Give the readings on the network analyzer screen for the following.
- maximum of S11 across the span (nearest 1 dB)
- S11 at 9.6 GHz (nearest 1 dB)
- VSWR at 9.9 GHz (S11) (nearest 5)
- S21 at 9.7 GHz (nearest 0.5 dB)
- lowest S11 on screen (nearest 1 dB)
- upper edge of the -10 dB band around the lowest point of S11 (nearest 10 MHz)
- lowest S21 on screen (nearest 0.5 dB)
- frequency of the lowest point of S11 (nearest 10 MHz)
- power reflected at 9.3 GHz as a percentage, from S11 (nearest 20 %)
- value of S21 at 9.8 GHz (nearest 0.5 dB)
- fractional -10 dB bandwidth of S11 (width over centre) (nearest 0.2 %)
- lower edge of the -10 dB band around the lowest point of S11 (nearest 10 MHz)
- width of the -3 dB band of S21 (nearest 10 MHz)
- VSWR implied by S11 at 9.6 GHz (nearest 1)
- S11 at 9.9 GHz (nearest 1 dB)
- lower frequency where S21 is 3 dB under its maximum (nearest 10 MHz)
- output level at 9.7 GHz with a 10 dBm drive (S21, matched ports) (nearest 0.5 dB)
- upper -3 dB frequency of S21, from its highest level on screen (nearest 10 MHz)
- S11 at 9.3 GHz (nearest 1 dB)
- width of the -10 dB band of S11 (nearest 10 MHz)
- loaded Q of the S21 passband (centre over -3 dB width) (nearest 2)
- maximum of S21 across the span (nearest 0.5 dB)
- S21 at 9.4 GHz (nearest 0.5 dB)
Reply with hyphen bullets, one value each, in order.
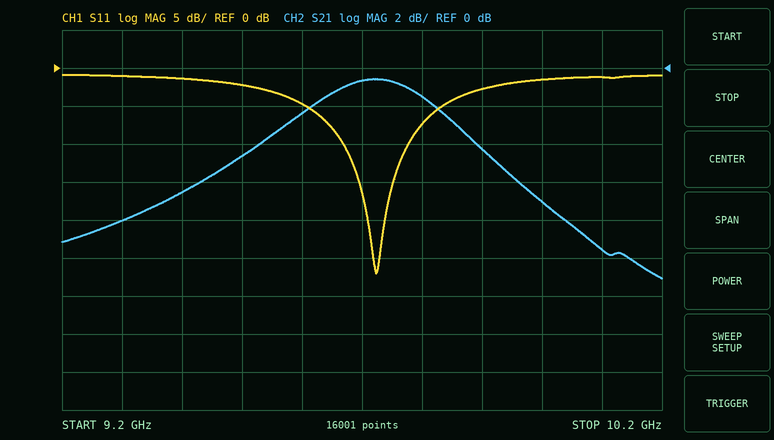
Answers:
- -1 dB
- -5 dB
- 5
- -0.5 dB
- -27 dB
- 9.78 GHz
- -11.0 dB
- 9.72 GHz
- 80 %
- -1.5 dB
- 1.2 %
- 9.67 GHz
- 330 MHz
- 4
- -3 dB
- 9.55 GHz
- 9.5 dBm
- 9.88 GHz
- -1 dB
- 110 MHz
- 30
- -0.5 dB
- -6.5 dB
